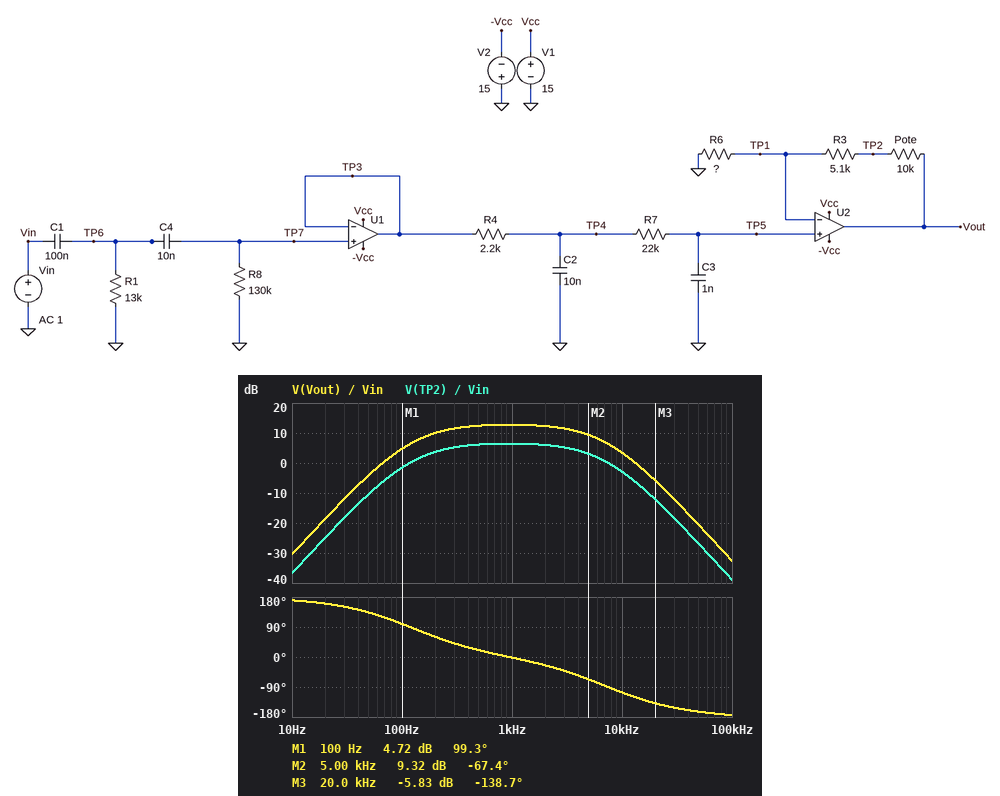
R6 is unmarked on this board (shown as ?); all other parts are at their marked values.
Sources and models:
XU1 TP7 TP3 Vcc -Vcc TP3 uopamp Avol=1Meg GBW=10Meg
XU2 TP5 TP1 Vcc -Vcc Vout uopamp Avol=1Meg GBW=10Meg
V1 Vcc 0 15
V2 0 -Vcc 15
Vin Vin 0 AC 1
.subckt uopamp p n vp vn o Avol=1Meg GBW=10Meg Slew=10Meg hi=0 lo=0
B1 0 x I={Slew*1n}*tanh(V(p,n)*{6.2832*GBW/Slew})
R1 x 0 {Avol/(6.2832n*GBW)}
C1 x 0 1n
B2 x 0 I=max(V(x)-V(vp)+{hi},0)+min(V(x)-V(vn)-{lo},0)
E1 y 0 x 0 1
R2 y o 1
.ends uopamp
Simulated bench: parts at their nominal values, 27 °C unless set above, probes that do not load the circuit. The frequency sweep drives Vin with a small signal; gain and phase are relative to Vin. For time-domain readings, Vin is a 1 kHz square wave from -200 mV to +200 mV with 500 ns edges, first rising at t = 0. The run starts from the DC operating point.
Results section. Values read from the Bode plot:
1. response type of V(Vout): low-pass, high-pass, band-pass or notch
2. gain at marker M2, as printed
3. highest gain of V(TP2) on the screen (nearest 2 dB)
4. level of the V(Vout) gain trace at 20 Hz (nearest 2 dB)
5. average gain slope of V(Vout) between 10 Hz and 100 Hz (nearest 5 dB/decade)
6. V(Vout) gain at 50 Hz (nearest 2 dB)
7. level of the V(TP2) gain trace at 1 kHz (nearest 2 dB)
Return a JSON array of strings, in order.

["band-pass", "9.32 dB", "6 dB", "-18 dB", "35 dB/decade", "-4 dB", "6 dB"]
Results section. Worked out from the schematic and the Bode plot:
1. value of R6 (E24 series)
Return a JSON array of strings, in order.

["4.3 kΩ"]
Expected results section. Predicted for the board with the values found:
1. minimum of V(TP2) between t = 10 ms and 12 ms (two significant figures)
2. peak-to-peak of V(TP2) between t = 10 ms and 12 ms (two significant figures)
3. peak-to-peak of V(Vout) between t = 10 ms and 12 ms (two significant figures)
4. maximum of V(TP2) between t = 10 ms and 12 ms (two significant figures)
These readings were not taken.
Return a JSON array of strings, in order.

["-510 mV", "1.0 V", "2.1 V", "510 mV"]
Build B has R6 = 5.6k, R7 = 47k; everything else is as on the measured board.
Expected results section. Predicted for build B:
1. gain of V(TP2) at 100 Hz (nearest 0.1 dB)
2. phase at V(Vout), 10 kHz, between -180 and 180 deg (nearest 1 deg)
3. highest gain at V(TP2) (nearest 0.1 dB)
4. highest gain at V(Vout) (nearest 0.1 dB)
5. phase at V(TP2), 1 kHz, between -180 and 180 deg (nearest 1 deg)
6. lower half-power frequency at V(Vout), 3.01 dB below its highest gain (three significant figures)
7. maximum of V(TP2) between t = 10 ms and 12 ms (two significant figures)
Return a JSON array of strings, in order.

["-2.7 dB", "-123 deg", "5.1 dB", "10.8 dB", "-10 deg", "184 Hz", "410 mV"]
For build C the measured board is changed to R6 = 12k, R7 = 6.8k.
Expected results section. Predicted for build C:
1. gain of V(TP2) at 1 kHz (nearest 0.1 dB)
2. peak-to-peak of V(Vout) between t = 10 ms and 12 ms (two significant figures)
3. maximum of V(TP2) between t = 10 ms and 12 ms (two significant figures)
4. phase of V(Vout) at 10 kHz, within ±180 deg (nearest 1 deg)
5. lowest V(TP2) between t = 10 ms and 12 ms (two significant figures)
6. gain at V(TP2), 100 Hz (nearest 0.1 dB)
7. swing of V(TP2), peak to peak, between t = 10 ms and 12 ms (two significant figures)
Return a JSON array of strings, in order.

["2.8 dB", "1.1 V", "340 mV", "-77 deg", "-340 mV", "-5.3 dB", "690 mV"]
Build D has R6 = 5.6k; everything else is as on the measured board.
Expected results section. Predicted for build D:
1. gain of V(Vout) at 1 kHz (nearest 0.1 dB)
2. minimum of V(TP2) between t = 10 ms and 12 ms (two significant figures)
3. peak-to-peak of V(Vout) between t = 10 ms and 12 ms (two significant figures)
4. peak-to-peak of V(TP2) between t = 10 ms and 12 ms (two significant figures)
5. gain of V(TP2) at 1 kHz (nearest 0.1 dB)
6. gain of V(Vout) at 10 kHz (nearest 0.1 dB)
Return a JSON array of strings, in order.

["11.0 dB", "-450 mV", "1.7 V", "890 mV", "5.3 dB", "1.7 dB"]
